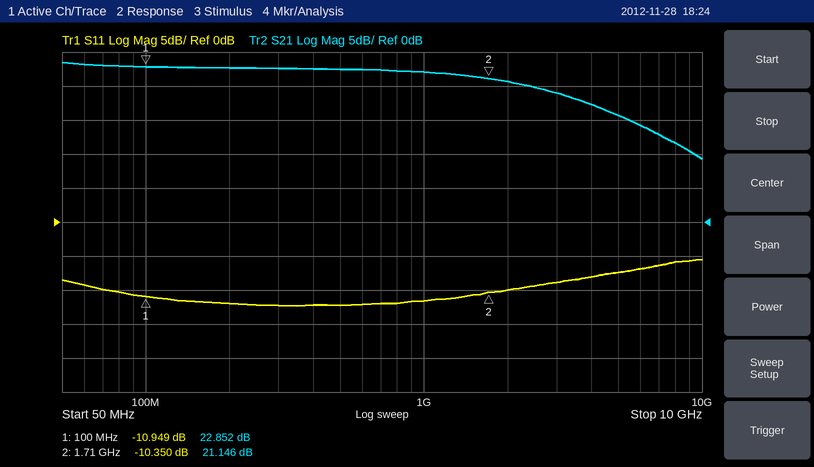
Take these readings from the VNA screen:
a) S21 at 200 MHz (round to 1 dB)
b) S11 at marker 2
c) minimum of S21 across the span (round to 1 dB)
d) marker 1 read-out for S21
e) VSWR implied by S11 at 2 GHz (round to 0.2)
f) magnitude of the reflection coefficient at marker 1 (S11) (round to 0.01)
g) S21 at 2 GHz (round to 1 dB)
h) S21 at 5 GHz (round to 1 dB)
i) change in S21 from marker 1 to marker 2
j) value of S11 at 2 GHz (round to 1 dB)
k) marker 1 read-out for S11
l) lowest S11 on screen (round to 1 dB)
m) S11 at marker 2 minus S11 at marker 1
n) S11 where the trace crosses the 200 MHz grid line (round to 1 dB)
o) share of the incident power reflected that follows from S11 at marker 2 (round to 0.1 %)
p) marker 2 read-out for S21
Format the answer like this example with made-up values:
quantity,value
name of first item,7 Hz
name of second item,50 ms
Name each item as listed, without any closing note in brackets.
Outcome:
quantity,value
S21 at 200 MHz,23 dB
S11 at marker 2,-10.350 dB
minimum of S21 across the span,9 dB
marker 1 read-out for S21,22.852 dB
VSWR implied by S11 at 2 GHz,2.0
magnitude of the reflection coefficient at marker 1 (S11),0.28
S21 at 2 GHz,21 dB
S21 at 5 GHz,16 dB
change in S21 from marker 1 to marker 2,-1.706 dB
value of S11 at 2 GHz,-10 dB
marker 1 read-out for S11,-10.949 dB
lowest S11 on screen,-12 dB
S11 at marker 2 minus S11 at marker 1,0.599 dB
S11 where the trace crosses the 200 MHz grid line,-12 dB
share of the incident power reflected that follows from S11 at marker 2,9.2 %
marker 2 read-out for S21,21.146 dB
